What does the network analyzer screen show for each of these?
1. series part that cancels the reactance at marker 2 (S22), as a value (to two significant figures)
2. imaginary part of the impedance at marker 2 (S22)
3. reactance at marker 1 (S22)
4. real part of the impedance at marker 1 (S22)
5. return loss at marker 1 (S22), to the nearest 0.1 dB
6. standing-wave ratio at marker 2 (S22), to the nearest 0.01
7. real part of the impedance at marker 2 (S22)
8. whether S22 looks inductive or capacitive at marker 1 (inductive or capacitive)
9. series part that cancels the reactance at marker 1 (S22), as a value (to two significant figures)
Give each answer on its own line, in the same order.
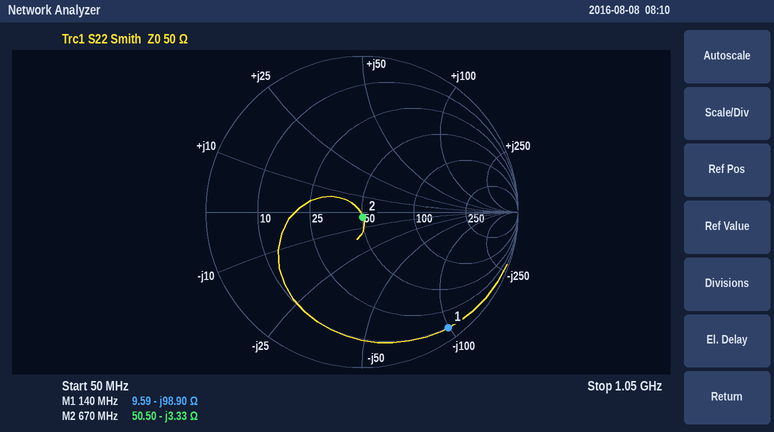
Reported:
790 pH
-3.33 Ω
-98.90 Ω
9.59 Ω
0.7 dB
1.07
50.50 Ω
capacitive
110 nH
